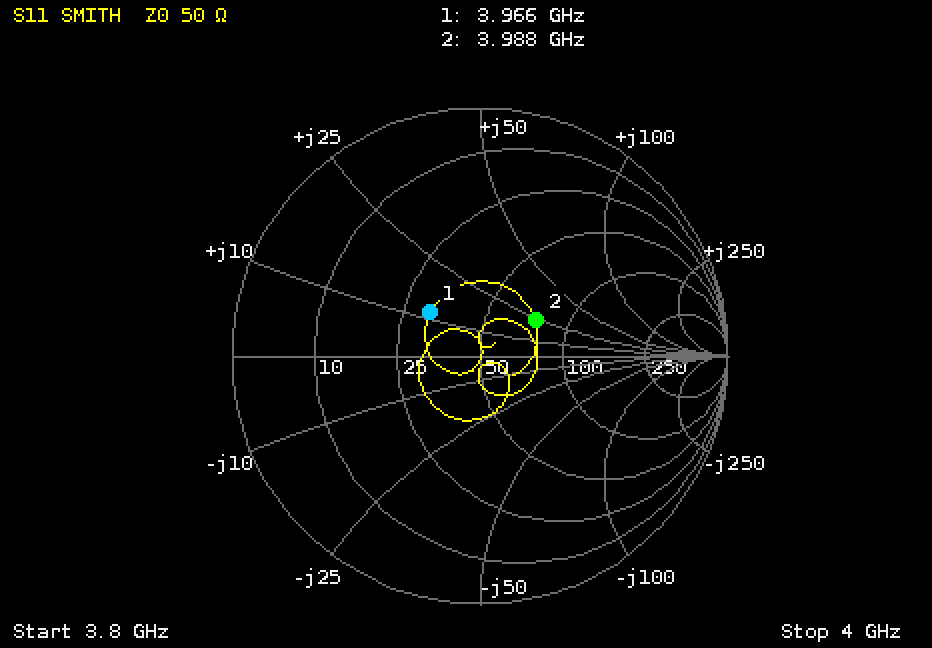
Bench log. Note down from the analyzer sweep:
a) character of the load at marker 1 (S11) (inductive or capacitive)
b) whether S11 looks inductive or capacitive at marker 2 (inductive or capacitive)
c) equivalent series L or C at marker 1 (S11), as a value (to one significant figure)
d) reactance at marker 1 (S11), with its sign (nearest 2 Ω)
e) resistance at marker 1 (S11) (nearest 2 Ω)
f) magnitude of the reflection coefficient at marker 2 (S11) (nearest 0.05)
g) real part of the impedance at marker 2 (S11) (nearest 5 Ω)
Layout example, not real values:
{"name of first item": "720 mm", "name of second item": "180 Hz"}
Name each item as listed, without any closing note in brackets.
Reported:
{"character of the load at marker 1 (S11)": "inductive", "whether S11 looks inductive or capacitive at marker 2": "inductive", "equivalent series L or C at marker 1 (S11), as a value": "500 pH", "reactance at marker 1 (S11), with its sign": "+12 Ω", "resistance at marker 1 (S11)": "32 Ω", "magnitude of the reflection coefficient at marker 2 (S11)": "0.25", "real part of the impedance at marker 2 (S11)": "75 Ω"}
